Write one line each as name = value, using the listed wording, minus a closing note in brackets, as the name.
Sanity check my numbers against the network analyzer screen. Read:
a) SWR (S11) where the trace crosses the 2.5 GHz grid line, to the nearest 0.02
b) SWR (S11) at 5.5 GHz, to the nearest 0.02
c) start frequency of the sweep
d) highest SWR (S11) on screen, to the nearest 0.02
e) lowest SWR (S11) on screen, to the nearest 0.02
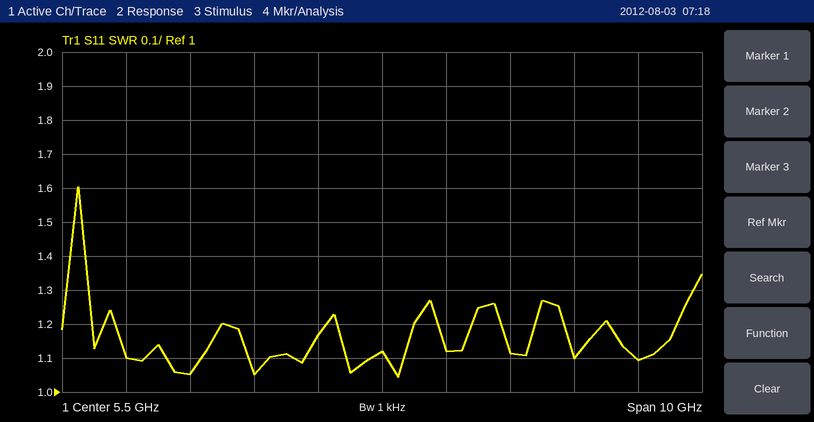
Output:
SWR (S11) where the trace crosses the 2.5 GHz grid line, to the nearest 0.02 = 1.06
SWR (S11) at 5.5 GHz, to the nearest 0.02 = 1.12
start frequency of the sweep = 500 MHz
highest SWR (S11) on screen, to the nearest 0.02 = 1.60
lowest SWR (S11) on screen, to the nearest 0.02 = 1.04
